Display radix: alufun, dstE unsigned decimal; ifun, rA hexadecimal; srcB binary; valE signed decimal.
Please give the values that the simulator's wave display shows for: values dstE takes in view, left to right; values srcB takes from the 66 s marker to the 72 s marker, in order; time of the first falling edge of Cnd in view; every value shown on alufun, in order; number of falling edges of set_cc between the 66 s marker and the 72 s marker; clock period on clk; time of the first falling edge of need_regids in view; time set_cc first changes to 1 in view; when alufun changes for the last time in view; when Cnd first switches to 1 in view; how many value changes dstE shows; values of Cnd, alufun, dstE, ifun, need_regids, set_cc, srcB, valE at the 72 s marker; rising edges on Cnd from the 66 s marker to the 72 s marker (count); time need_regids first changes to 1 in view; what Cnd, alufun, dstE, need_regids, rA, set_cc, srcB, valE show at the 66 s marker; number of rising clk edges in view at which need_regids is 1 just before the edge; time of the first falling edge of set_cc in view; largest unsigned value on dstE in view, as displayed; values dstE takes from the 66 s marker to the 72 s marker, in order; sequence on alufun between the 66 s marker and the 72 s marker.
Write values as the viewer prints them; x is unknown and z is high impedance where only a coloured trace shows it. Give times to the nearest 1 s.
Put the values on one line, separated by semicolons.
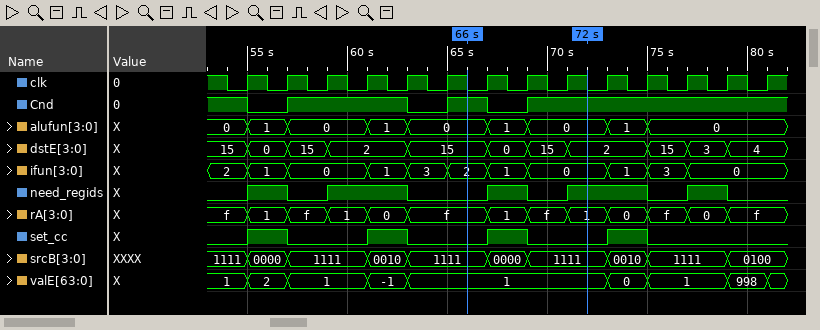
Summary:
15, 0, 15, 2, 15, 0, 15, 2, 15, 3, 4; 1111, 0000, 1111; 55 s; 0, 1, 0, 1, 0, 1, 0, 1, 0; 1; 2 s; 57 s; 55 s; 75 s; 57 s; 10; Cnd=1, alufun=0, dstE=2, ifun=0, need_regids=1, set_cc=0, srcB=1111, valE=1; 1; 55 s; Cnd=1, alufun=0, dstE=15, need_regids=0, rA=f, set_cc=0, srcB=1111, valE=1; 7; 57 s; 15; 15, 0, 15, 2; 0, 1, 0
